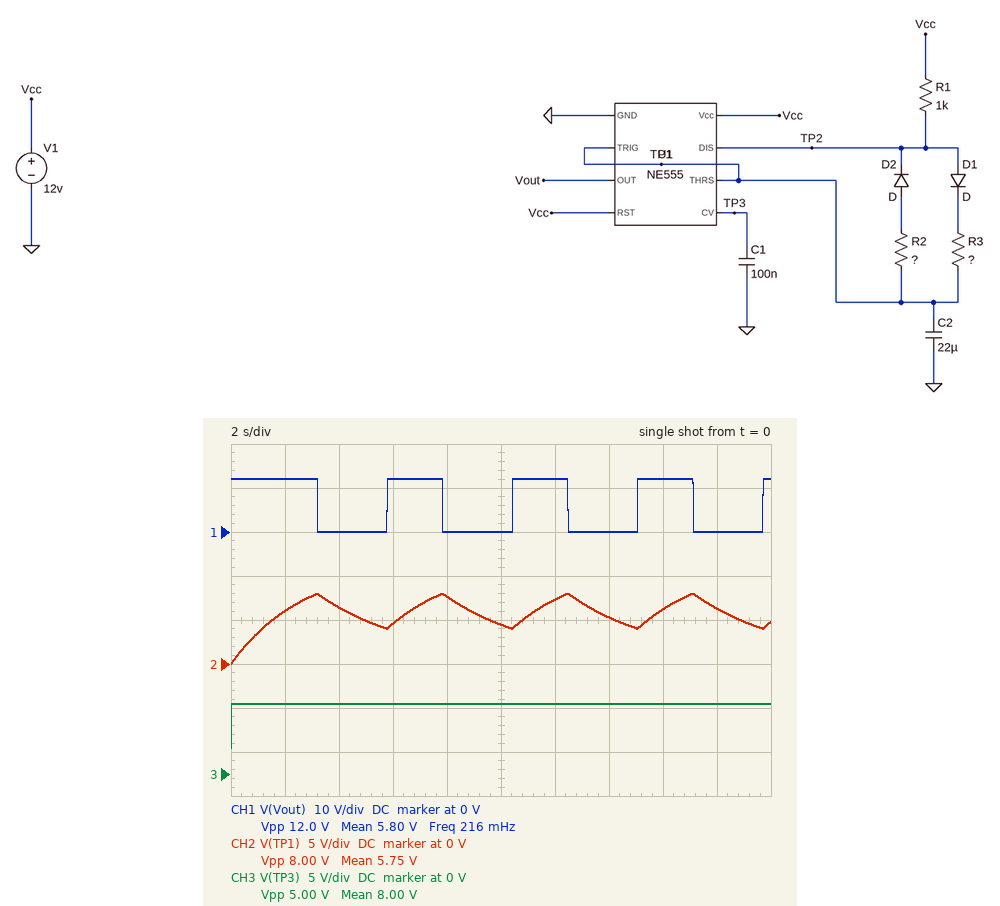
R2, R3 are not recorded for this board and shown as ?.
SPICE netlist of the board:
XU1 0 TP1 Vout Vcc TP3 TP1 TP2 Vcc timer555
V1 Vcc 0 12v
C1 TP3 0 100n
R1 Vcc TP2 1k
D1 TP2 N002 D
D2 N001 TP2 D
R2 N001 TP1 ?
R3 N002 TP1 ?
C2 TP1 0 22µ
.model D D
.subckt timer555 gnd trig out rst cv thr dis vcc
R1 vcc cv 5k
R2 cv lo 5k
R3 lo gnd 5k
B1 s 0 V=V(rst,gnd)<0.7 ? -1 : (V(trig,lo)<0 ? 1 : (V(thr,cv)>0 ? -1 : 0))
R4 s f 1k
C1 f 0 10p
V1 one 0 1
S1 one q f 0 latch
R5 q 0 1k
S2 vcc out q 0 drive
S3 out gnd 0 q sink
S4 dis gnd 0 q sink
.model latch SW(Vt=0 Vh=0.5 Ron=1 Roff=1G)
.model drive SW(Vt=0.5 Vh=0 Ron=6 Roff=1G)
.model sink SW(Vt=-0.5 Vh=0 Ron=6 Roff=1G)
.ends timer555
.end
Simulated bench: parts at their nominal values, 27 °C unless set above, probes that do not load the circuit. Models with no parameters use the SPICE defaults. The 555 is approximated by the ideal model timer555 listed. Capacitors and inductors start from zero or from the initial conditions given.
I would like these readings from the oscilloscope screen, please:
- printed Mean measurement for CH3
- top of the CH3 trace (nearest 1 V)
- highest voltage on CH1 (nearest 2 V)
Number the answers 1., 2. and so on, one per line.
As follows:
1. 8.00 V
2. 8 V
3. 12 V
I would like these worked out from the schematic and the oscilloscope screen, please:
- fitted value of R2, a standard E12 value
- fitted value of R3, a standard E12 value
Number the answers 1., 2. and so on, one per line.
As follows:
1. 150 kΩ
2. 120 kΩ
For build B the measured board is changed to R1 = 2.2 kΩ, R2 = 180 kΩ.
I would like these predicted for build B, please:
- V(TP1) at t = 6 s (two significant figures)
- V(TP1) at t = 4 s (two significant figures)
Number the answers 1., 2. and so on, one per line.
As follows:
1. 4.3 V
2. 6.7 V
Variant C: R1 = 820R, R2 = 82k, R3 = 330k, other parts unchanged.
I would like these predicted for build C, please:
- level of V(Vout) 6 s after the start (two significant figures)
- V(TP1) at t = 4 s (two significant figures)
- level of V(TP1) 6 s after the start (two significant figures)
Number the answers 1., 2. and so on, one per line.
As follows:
1. 12 V
2. 4.8 V
3. 6.4 V
